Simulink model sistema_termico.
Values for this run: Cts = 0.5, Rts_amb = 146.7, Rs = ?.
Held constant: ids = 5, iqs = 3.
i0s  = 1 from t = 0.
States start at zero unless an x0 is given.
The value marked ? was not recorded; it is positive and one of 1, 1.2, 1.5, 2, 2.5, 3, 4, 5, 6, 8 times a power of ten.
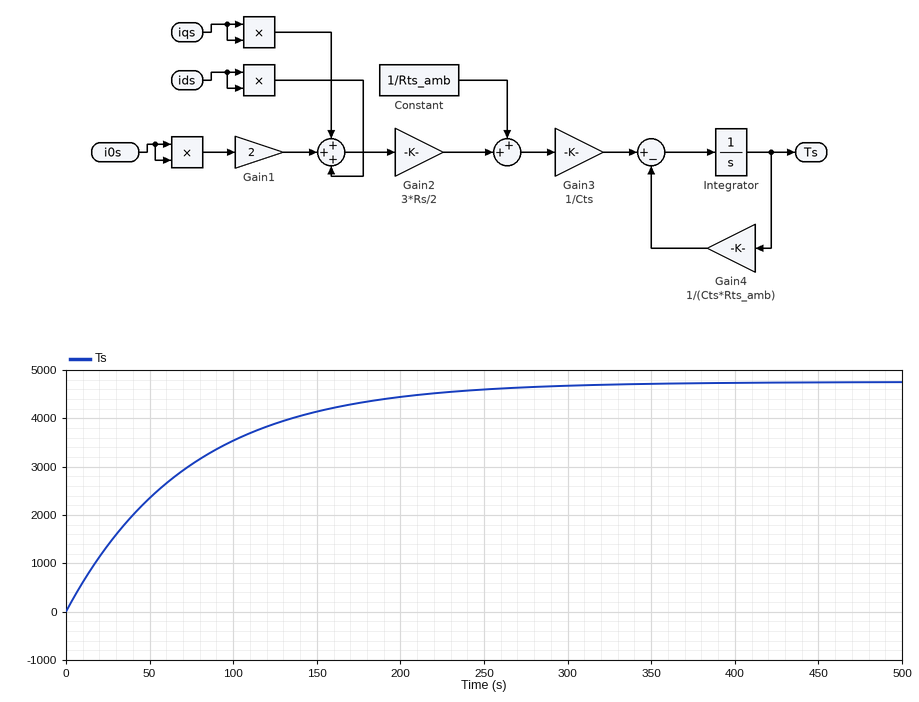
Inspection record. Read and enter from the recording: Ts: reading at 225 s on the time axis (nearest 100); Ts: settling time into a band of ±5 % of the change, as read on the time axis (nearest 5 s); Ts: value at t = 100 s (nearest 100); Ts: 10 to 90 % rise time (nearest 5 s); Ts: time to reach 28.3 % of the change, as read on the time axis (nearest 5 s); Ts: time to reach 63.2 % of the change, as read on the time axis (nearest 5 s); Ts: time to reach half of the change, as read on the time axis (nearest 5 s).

4500
220 s
3500
160 s
25 s
75 s
50 s
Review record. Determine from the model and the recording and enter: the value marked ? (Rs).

0.6
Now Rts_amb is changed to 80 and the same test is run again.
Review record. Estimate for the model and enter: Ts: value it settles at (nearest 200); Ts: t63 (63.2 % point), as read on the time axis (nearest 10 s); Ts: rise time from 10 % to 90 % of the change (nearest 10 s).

2600
40 s
90 s
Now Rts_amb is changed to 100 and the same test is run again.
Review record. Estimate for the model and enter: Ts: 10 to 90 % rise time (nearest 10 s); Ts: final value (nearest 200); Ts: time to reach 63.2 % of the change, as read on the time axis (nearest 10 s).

110 s
3200
50 s
